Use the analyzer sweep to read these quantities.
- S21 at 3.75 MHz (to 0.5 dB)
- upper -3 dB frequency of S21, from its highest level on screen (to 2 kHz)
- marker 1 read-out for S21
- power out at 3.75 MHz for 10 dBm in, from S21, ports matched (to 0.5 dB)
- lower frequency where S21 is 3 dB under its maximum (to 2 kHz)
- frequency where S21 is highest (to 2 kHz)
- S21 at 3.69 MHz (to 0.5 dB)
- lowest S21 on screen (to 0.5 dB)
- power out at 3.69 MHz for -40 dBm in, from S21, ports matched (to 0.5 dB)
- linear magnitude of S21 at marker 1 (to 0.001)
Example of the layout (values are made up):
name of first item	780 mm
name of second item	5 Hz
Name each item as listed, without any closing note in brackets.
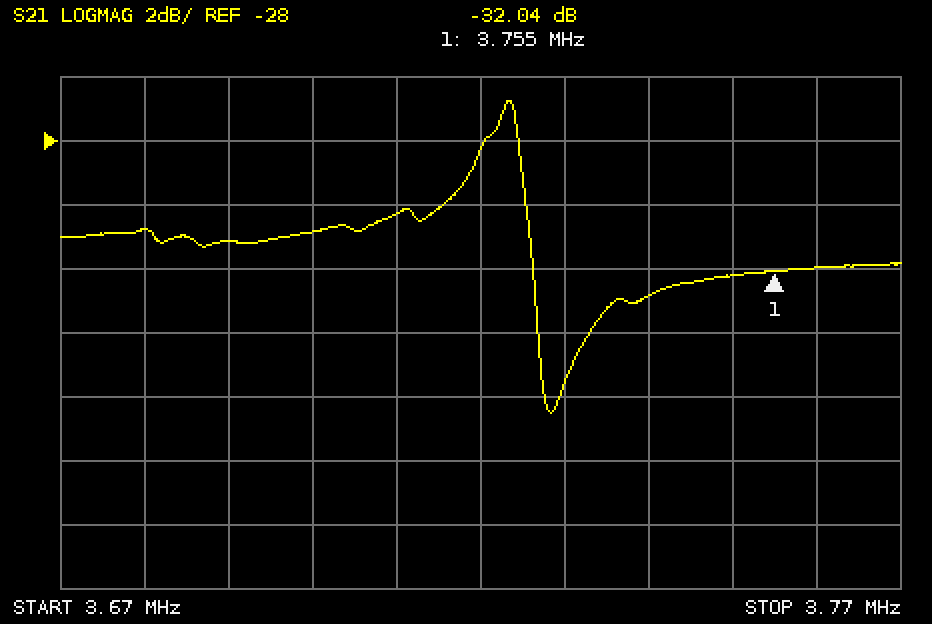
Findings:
S21 at 3.75 MHz	-32.0 dB
upper -3 dB frequency of S21, from its highest level on screen	3.726 MHz
marker 1 read-out for S21	-32.04 dB
power out at 3.75 MHz for 10 dBm in, from S21, ports matched	-22.0 dBm
lower frequency where S21 is 3 dB under its maximum	3.716 MHz
frequency where S21 is highest	3.724 MHz
S21 at 3.69 MHz	-31.0 dB
lowest S21 on screen	-36.5 dB
power out at 3.69 MHz for -40 dBm in, from S21, ports matched	-71.0 dBm
linear magnitude of S21 at marker 1	0.025
